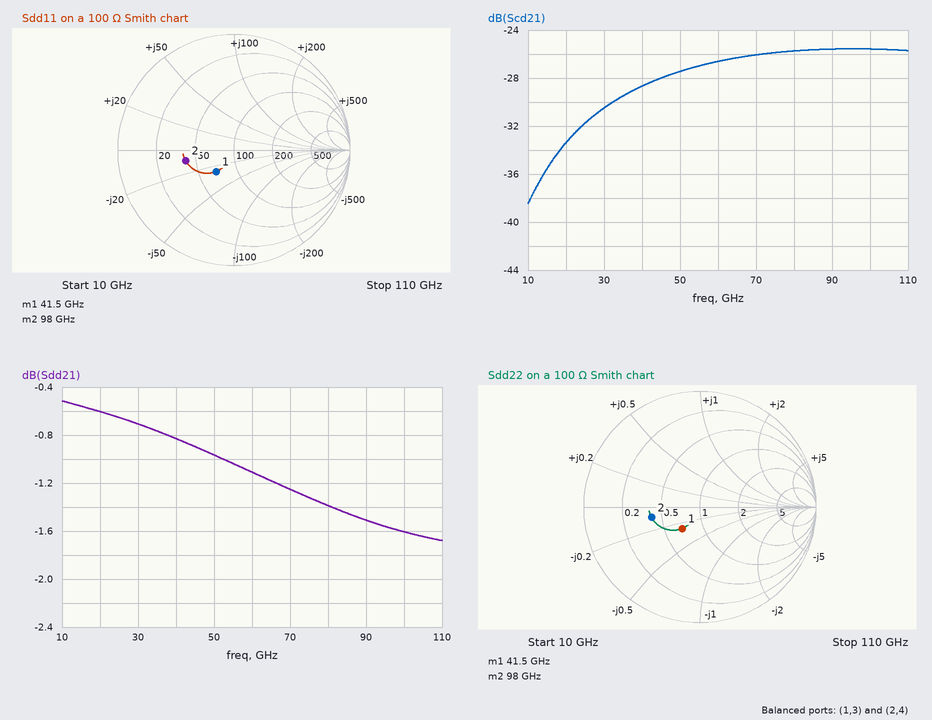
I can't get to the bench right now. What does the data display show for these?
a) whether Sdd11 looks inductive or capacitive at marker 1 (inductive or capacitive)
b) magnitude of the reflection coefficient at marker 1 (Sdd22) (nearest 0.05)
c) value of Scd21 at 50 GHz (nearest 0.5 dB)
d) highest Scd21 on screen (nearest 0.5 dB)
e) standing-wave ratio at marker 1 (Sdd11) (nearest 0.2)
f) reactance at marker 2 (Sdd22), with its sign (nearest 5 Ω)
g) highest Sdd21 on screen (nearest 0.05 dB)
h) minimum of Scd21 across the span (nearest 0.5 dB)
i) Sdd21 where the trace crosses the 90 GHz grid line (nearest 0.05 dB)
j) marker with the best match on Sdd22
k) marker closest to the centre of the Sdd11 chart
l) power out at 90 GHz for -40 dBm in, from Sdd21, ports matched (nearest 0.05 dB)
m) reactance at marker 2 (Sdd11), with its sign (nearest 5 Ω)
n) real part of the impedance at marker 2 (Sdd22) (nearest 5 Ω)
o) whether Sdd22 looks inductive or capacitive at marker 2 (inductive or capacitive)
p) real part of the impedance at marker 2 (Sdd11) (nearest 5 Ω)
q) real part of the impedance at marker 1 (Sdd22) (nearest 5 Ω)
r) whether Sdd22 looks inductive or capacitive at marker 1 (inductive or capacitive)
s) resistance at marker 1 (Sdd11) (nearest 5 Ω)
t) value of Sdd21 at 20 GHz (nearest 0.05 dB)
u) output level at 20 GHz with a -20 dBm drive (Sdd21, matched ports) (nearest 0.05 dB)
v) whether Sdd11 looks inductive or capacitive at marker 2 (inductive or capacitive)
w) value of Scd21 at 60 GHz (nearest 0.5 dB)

capacitive
0.25
-27.5 dB
-25.5 dB
1.6
-10 Ω
-0.50 dB
-38.5 dB
-1.50 dB
marker 1
marker 1
-41.50 dBm
-10 Ω
40 Ω
capacitive
40 Ω
70 Ω
capacitive
70 Ω
-0.60 dB
-20.60 dBm
capacitive
-26.5 dB
